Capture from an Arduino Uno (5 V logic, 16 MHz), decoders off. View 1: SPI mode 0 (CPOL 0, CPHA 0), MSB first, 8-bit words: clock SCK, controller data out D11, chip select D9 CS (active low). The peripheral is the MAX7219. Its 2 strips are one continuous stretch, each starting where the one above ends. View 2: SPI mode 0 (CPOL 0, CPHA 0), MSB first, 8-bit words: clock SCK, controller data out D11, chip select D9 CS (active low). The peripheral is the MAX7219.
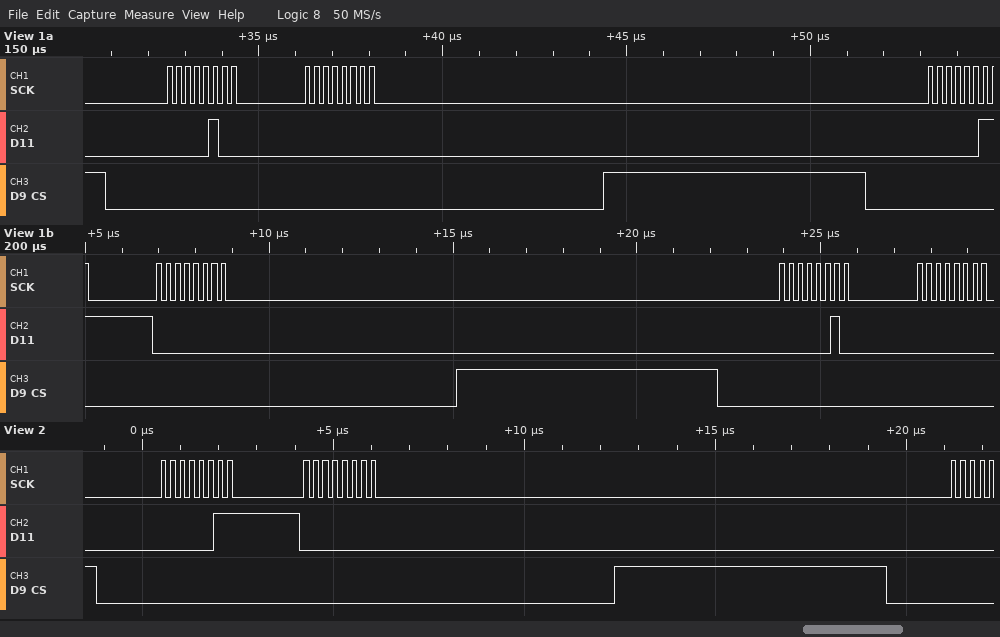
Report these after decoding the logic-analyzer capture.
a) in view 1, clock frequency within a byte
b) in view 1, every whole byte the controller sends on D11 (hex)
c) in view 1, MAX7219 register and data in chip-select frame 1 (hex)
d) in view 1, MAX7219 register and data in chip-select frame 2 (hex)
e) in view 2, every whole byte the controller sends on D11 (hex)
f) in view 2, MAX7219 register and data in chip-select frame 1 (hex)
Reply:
4 MHz
0x04 0x00 0x03 0x00 0x02 0x00
register 0x4, data 0x00
register 0x3, data 0x00
03 00
register 0x3, data 0x00
